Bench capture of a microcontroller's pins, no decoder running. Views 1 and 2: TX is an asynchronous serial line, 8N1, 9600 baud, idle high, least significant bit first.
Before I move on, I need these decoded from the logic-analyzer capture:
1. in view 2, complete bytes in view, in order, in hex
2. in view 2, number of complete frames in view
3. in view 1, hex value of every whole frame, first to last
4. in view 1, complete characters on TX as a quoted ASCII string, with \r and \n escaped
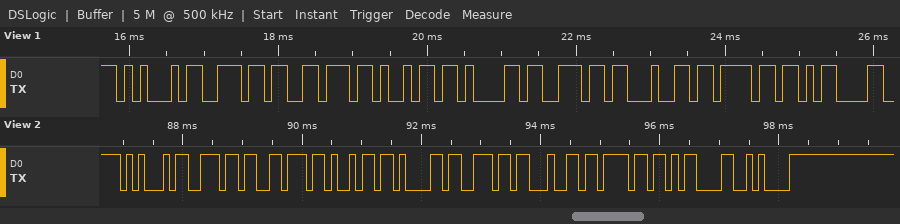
0x45 0x6E 0x76 0x69 0x61 0x6E 0x64 0x6F 0x0D 0x0A
10
45 6E 76 69 61 6E 64 6F 0D
"Enviando\r"
